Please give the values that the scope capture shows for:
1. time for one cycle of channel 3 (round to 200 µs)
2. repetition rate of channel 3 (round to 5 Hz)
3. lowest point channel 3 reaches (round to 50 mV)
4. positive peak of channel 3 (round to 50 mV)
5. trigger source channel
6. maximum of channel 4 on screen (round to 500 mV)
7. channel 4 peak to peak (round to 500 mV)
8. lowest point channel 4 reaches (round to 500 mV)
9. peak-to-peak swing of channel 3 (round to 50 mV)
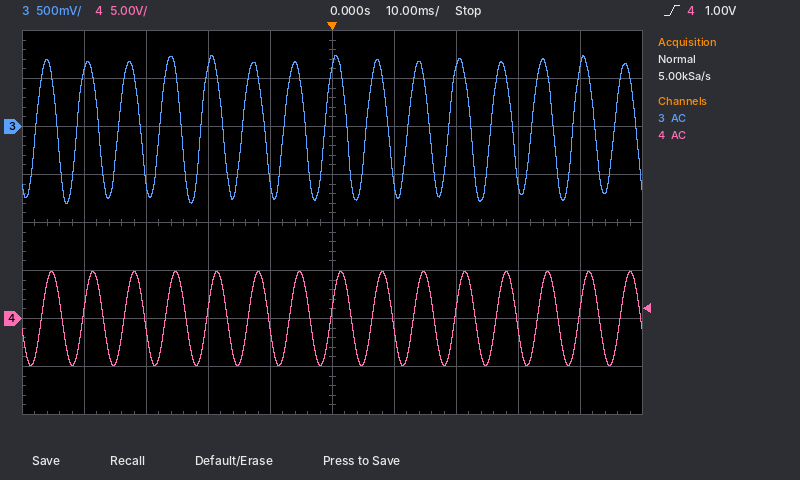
6.6 ms
150 Hz
-800 mV
750 mV
channel 4
5.0 V
10.0 V
-5.0 V
1.55 V
